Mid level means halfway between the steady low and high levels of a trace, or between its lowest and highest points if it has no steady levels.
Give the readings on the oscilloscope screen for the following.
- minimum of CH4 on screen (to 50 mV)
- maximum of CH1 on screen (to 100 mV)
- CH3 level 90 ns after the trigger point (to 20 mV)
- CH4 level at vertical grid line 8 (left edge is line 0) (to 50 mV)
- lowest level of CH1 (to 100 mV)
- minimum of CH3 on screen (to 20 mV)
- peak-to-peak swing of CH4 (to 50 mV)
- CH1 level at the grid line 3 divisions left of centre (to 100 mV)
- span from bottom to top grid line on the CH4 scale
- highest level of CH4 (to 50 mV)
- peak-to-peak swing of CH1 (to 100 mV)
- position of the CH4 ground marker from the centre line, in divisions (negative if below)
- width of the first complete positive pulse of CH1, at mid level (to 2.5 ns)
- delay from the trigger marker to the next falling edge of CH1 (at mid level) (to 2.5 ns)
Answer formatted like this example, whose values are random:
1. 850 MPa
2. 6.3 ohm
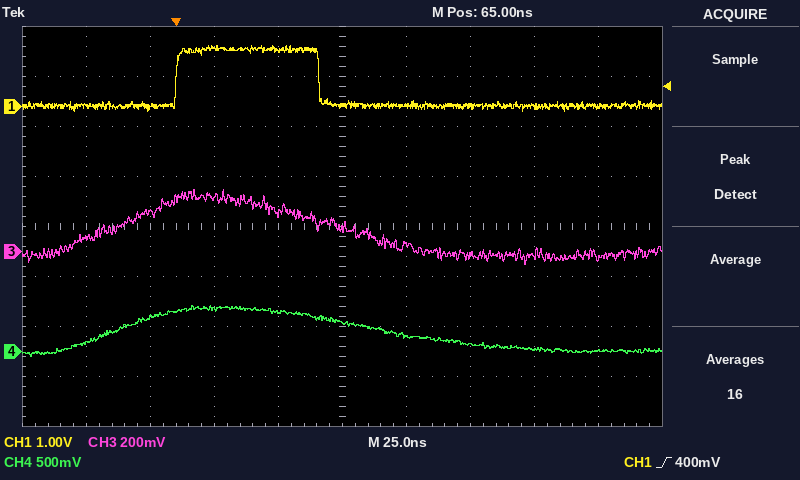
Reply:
1. -50 mV
2. 1.2 V
3. 20 mV
4. 0 mV
5. -100 mV
6. -60 mV
7. 500 mV
8. 0.0 V
9. 4 V
10. 450 mV
11. 1.3 V
12. -2.5 div
13. 55.0 ns
14. 55.0 ns
